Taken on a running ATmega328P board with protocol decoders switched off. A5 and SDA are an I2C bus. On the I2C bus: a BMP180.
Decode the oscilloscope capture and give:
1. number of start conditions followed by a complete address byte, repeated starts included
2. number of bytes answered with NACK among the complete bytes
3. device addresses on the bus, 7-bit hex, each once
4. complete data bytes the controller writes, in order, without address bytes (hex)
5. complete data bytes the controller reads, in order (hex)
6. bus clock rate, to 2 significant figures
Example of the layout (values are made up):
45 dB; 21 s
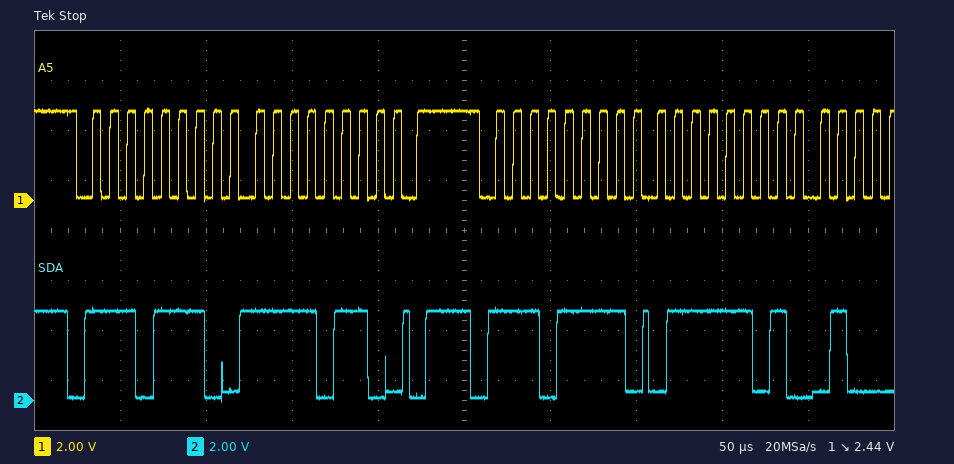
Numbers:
2; 0; 0x77; F6; 7D; 100 kHz
